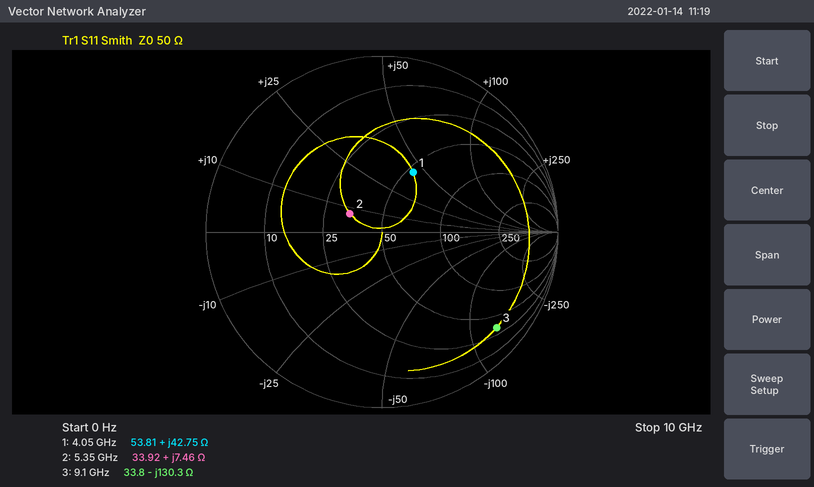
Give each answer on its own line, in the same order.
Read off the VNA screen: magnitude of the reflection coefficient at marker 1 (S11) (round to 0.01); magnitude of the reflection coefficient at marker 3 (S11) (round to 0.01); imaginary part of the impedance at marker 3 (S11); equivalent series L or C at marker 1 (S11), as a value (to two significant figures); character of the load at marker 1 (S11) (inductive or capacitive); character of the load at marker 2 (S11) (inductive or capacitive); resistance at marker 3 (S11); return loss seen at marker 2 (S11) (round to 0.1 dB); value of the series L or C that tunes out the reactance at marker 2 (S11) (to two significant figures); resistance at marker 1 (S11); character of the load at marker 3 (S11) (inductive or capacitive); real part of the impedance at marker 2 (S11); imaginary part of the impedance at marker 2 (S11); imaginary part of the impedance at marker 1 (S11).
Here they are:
0.38
0.85
-130.3 Ω
1.7 nH
inductive
inductive
33.8 Ω
13.5 dB
4.0 pF
53.81 Ω
capacitive
33.92 Ω
+7.46 Ω
+42.75 Ω
